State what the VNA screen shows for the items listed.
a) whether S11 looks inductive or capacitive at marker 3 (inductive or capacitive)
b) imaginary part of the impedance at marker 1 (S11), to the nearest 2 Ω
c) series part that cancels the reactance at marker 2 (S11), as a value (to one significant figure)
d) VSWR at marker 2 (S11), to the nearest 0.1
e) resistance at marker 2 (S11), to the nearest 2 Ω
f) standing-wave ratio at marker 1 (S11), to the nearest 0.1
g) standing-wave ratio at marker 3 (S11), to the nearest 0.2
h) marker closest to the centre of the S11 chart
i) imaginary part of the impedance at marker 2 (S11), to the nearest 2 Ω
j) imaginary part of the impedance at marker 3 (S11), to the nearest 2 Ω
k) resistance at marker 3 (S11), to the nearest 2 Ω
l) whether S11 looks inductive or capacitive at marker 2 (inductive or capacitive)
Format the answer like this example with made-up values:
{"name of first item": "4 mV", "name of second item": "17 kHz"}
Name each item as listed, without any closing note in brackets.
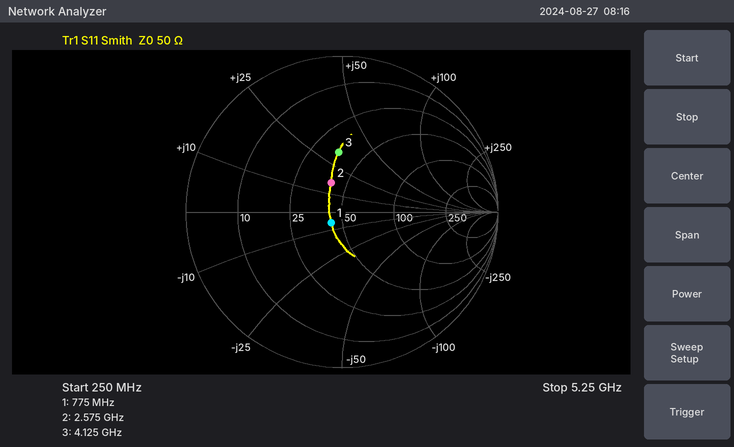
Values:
{"whether S11 looks inductive or capacitive at marker 3": "inductive", "imaginary part of the impedance at marker 1 (S11), to the nearest 2 Ω": "-6 Ω", "series part that cancels the reactance at marker 2 (S11), as a value": "4 pF", "VSWR at marker 2 (S11), to the nearest 0.1": "1.5", "resistance at marker 2 (S11), to the nearest 2 Ω": "40 Ω", "standing-wave ratio at marker 1 (S11), to the nearest 0.1": "1.2", "standing-wave ratio at marker 3 (S11), to the nearest 0.2": "2.2", "marker closest to the centre of the S11 chart": "marker 1", "imaginary part of the impedance at marker 2 (S11), to the nearest 2 Ω": "+16 Ω", "imaginary part of the impedance at marker 3 (S11), to the nearest 2 Ω": "+32 Ω", "resistance at marker 3 (S11), to the nearest 2 Ω": "36 Ω", "whether S11 looks inductive or capacitive at marker 2": "inductive"}
